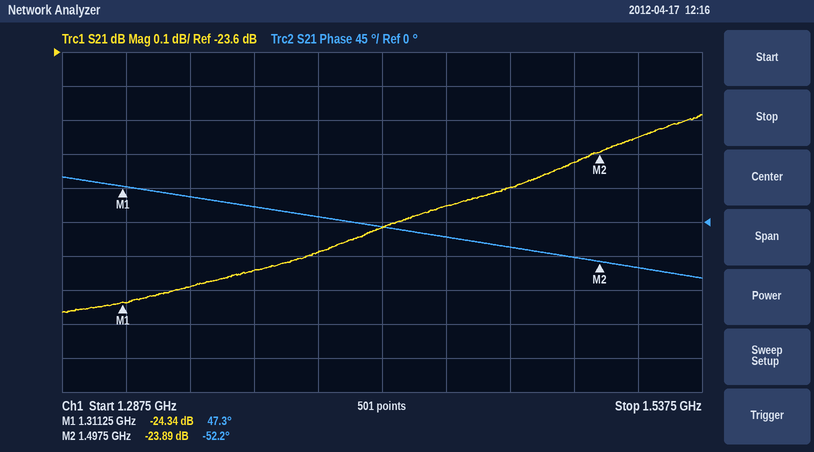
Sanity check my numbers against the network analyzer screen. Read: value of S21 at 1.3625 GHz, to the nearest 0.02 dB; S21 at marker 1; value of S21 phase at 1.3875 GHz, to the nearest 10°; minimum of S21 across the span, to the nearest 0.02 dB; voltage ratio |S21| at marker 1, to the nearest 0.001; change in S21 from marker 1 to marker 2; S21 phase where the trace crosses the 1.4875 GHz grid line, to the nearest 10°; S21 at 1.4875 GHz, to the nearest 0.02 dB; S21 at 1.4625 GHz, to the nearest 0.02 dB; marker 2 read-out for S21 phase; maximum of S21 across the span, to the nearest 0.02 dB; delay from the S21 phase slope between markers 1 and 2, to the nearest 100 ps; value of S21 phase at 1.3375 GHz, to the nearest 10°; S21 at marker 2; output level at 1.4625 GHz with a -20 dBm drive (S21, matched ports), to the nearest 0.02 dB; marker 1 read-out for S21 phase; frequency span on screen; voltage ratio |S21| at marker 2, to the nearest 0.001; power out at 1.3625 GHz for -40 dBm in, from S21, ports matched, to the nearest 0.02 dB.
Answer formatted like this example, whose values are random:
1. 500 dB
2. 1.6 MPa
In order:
1. -24.24 dB
2. -24.34 dB
3. 10°
4. -24.36 dB
5. 0.061
6. 0.45 dB
7. -50°
8. -23.92 dB
9. -24.00 dB
10. -52.2°
11. -23.78 dB
12. 1.5 ns
13. 30°
14. -23.89 dB
15. -44.00 dBm
16. 47.3°
17. 250 MHz
18. 0.064
19. -64.24 dBm
